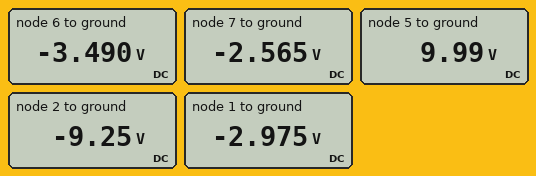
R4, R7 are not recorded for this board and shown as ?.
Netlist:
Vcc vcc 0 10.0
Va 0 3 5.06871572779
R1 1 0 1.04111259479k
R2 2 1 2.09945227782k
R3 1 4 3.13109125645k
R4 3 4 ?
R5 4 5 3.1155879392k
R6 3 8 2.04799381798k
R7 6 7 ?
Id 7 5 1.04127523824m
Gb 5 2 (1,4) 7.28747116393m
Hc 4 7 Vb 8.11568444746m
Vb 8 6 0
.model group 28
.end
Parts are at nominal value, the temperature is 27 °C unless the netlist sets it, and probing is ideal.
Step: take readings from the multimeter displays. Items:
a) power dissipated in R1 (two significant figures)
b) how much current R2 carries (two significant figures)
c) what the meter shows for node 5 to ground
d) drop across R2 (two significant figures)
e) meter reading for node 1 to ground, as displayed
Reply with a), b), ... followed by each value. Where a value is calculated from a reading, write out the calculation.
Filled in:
a) (0 V - (-2.975 V))^2 / 1.041 kΩ = 8.5 mW
b) (-2.975 V - (-9.25 V)) / 2.099 kΩ = 3.0 mA
c) 9.99 V
d) -2.975 V - (-9.25 V) = 6.3 V
e) -2.975 V
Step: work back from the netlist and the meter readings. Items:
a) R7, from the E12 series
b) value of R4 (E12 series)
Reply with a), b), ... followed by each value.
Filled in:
a) 1.2 kΩ
b) 1.2 kΩ
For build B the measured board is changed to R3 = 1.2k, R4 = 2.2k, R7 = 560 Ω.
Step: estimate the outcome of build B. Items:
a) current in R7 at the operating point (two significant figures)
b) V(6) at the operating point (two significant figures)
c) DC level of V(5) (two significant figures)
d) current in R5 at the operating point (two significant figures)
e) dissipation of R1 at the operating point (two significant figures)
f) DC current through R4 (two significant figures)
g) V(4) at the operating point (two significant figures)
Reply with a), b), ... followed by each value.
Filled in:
a) 1.1 mA
b) -2.8 V
c) 9.7 V
d) 3.8 mA
e) 6.2 mW
f) 1.3 mA
g) -2.2 V
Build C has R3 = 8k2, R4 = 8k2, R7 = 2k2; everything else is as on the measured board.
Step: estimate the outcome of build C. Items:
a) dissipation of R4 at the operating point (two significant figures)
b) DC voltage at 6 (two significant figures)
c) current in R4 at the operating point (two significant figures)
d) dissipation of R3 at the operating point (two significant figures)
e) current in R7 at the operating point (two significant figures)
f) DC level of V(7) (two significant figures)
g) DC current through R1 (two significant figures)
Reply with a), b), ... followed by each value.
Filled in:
a) 1.8 mW
b) -3.2 V
c) 470 µA
d) 4.5 µW
e) 900 µA
f) -1.2 V
g) 1.4 mA
